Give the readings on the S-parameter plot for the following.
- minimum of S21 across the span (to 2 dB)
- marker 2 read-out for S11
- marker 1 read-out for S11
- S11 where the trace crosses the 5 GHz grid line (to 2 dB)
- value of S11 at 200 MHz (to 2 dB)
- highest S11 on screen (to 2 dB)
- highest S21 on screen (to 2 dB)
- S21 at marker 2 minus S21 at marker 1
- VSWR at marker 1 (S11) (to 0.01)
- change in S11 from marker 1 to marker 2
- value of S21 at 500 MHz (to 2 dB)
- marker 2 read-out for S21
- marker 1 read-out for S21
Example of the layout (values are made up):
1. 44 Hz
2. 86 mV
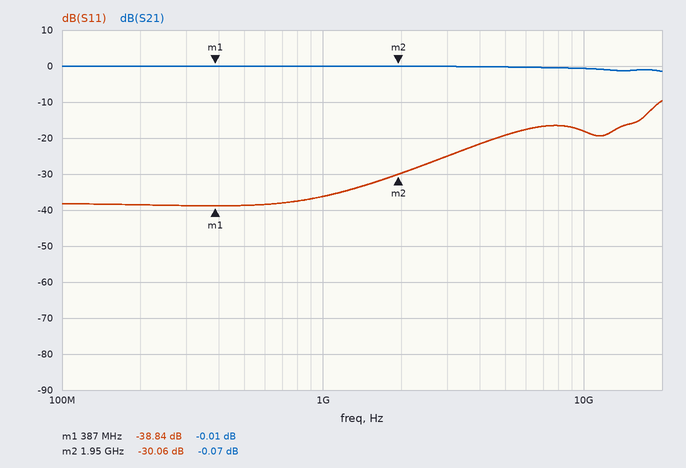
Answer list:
1. -2 dB
2. -30.06 dB
3. -38.84 dB
4. -20 dB
5. -38 dB
6. -10 dB
7. 0 dB
8. -0.06 dB
9. 1.02
10. 8.78 dB
11. 0 dB
12. -0.07 dB
13. -0.01 dB
